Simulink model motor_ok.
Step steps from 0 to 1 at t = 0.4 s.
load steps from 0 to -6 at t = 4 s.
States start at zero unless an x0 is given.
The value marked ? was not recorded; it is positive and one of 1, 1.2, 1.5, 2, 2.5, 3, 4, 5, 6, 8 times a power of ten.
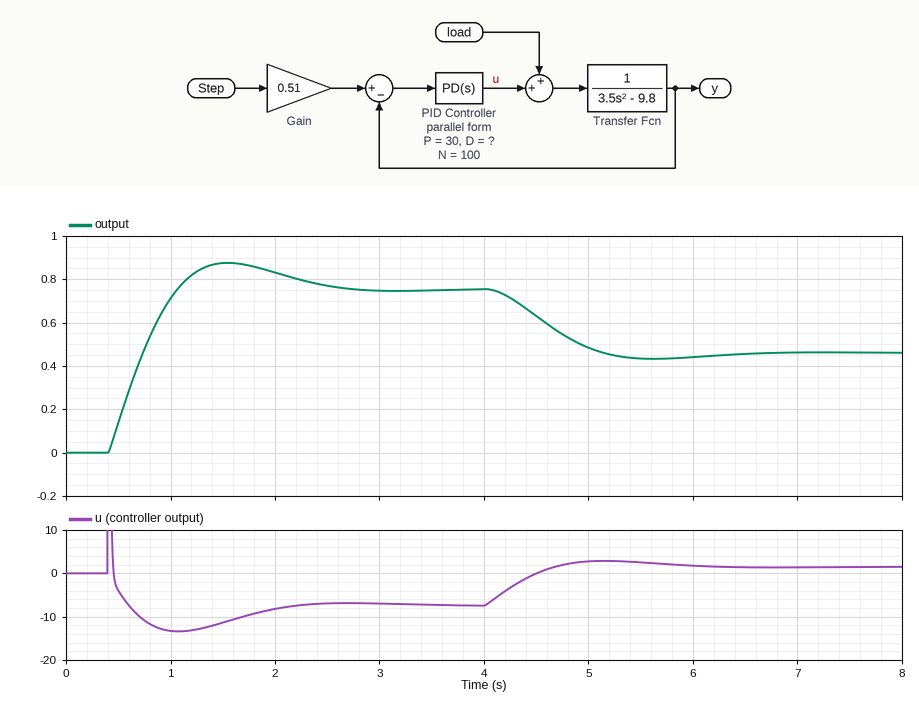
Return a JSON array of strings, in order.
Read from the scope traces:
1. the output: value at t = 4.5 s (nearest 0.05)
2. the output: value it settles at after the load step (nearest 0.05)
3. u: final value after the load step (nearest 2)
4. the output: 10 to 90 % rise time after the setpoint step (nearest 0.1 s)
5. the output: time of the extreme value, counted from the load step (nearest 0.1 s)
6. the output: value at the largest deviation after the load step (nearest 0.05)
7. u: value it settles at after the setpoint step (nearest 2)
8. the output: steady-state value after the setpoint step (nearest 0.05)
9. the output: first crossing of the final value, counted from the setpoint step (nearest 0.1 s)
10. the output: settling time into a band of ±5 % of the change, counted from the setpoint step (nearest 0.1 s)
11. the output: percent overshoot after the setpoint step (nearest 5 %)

["0.65", "0.45", "2", "0.5 s", "1.6 s", "0.45", "-8", "0.75", "0.7 s", "1.9 s", "15 %"]
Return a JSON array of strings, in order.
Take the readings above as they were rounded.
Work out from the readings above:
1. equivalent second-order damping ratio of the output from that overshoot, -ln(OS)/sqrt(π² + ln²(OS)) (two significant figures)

["0.52"]
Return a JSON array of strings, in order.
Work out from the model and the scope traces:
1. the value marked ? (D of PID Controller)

["10"]
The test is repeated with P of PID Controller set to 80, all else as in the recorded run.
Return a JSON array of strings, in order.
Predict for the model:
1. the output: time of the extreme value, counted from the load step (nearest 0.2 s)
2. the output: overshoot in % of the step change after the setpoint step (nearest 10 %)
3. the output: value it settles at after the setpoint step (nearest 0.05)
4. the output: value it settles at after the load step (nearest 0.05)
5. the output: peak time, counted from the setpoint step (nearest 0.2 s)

["0.8 s", "40 %", "0.60", "0.50", "0.6 s"]
